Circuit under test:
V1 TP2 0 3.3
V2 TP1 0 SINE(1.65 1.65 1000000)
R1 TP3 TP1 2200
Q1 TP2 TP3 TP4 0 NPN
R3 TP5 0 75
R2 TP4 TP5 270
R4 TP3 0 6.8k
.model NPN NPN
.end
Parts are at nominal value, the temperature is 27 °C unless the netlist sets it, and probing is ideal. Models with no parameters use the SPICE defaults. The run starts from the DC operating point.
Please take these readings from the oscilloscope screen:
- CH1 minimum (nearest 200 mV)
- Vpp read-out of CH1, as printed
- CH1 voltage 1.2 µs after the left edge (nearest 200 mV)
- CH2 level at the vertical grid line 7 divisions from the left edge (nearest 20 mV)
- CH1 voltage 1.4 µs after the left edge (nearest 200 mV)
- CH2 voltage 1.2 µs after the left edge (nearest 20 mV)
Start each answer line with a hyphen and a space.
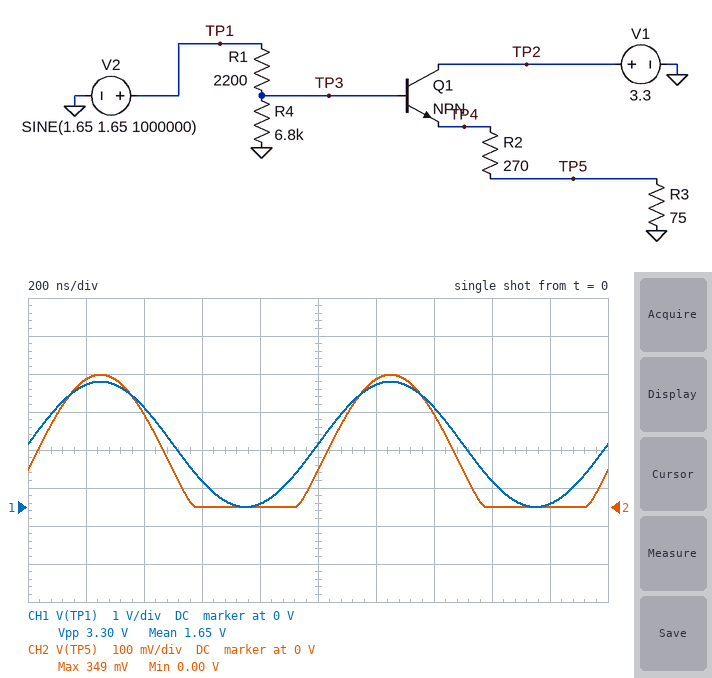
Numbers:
- 0 V
- 3.30 V
- 3.2 V
- 240 mV
- 2.6 V
- 340 mV
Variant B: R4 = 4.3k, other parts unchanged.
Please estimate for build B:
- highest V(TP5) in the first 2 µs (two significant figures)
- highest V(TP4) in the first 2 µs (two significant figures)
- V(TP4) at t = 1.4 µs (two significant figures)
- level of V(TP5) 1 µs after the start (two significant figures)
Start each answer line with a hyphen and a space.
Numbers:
- 290 mV
- 1.3 V
- 900 mV
- 67 mV
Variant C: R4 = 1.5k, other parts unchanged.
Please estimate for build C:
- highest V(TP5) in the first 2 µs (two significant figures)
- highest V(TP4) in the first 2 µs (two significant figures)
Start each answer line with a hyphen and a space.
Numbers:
- 120 mV
- 540 mV
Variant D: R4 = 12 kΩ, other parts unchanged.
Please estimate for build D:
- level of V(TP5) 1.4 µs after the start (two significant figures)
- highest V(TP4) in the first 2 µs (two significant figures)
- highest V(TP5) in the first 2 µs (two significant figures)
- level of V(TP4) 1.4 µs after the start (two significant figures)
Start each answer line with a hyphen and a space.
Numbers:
- 290 mV
- 1.9 V
- 410 mV
- 1.3 V
